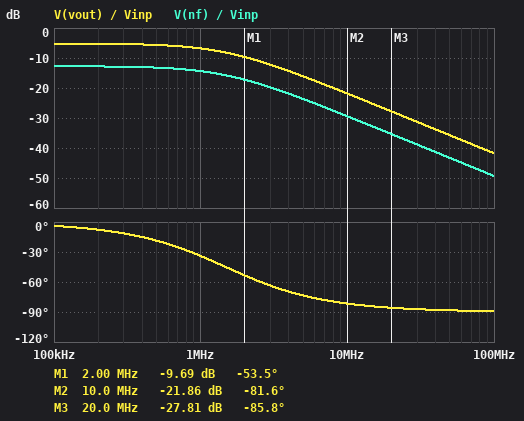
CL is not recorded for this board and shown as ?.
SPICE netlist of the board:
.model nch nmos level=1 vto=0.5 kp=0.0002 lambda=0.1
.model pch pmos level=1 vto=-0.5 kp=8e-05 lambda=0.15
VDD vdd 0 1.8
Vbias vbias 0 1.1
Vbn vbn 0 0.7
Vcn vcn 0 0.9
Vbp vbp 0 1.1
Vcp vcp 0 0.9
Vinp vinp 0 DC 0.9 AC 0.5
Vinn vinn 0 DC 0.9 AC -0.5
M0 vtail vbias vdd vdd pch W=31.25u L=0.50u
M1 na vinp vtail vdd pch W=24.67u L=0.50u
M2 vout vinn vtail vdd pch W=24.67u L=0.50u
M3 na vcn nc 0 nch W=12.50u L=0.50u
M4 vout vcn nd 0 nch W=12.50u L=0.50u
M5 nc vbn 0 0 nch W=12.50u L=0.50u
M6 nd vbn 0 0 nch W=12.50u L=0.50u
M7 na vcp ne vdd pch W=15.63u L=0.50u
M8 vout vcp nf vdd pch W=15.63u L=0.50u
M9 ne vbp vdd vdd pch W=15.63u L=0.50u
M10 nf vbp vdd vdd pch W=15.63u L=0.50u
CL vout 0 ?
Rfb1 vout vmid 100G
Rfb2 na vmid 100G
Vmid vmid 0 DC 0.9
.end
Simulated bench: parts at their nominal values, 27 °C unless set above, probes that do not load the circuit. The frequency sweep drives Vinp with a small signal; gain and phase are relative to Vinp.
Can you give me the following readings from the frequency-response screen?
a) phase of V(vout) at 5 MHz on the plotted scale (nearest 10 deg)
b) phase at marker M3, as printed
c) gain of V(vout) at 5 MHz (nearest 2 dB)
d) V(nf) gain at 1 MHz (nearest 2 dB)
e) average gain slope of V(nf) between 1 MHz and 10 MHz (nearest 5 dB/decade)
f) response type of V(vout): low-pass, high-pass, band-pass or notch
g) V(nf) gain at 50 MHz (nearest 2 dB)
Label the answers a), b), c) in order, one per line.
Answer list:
a) -70 deg
b) -85.8 deg
c) -16 dB
d) -14 dB
e) -15 dB/decade
f) low-pass
g) -44 dB
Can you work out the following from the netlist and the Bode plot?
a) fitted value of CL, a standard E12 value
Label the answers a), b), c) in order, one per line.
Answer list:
a) 6.8 pF
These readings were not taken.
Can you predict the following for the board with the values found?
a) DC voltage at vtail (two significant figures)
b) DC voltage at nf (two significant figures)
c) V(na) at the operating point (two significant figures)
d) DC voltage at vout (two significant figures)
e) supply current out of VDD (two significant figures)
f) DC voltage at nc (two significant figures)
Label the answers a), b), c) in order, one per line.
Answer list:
a) 1.6 V
b) 1.6 V
c) 1.5 V
d) 1.5 V
e) 200 µA
f) 210 mV
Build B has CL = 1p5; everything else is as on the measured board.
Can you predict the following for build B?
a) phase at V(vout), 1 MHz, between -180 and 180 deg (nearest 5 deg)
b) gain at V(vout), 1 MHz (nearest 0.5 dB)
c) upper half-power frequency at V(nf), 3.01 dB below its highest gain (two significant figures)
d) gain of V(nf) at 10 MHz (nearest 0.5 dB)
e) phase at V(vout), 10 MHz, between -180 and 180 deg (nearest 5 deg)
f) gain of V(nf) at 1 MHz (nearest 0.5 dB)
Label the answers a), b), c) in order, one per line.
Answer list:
a) -10 deg
b) -5.5 dB
c) 6.7 MHz
d) -18.0 dB
e) -55 deg
f) -13.0 dB
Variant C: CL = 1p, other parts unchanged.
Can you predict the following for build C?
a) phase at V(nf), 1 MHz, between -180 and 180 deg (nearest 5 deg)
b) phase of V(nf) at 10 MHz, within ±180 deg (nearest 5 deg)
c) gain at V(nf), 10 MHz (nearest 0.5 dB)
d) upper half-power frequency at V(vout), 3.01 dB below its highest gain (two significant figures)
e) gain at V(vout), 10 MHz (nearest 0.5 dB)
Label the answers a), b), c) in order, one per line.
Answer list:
a) -5 deg
b) -45 deg
c) -15.5 dB
d) 10 MHz
e) -8.0 dB
